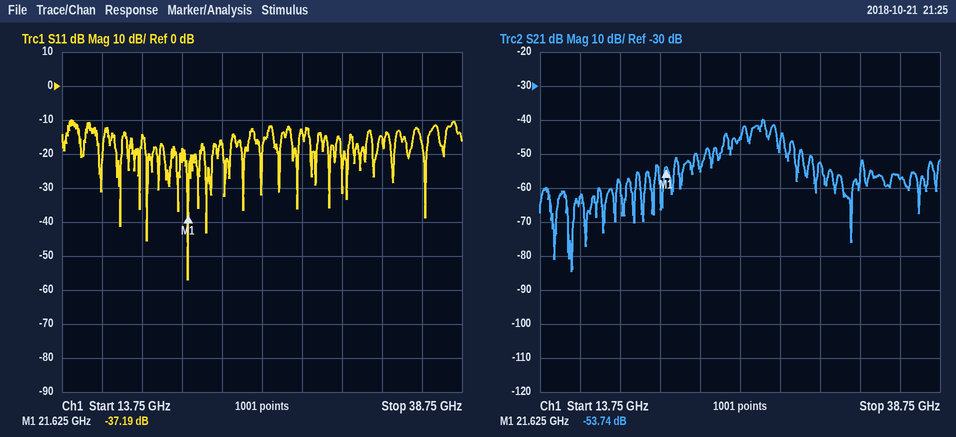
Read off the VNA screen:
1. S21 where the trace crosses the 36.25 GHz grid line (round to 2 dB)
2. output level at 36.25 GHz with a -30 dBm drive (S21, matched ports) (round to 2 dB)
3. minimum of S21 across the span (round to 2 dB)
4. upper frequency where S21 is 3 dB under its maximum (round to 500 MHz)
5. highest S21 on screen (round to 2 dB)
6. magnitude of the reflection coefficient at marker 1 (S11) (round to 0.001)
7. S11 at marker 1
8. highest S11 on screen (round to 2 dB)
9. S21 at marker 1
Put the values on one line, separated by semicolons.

-58 dB; -88 dBm; -84 dB; 28.0 GHz; -40 dB; 0.014; -37.19 dB; -10 dB; -53.74 dB
